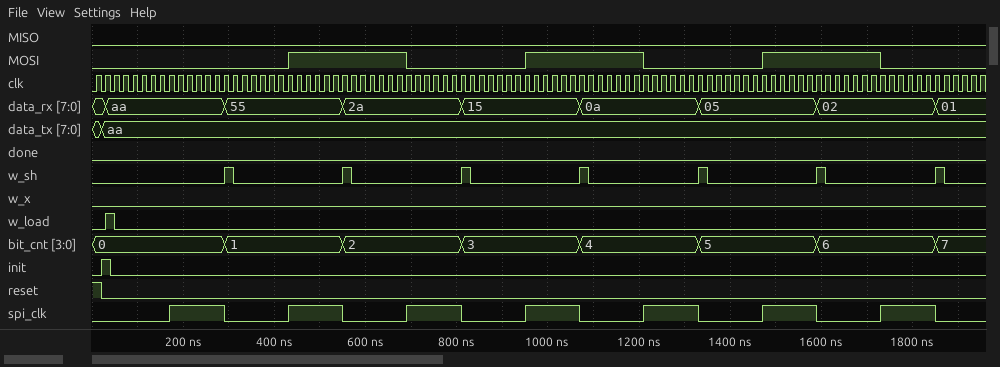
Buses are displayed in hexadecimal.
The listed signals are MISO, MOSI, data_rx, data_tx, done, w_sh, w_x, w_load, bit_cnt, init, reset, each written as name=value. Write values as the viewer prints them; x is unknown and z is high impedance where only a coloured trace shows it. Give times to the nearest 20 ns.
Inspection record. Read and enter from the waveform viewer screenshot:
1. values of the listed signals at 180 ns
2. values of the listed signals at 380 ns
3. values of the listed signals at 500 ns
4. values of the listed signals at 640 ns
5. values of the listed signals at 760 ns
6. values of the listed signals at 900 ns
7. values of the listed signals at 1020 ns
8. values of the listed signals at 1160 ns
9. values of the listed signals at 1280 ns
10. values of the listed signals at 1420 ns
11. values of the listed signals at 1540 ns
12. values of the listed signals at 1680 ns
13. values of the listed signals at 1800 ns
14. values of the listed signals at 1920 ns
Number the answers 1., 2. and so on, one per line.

1. MISO=0, MOSI=0, data_rx=aa, data_tx=aa, done=0, w_sh=0, w_x=0, w_load=0, bit_cnt=0, init=0, reset=0
2. MISO=0, MOSI=0, data_rx=55, data_tx=aa, done=0, w_sh=0, w_x=0, w_load=0, bit_cnt=1, init=0, reset=0
3. MISO=0, MOSI=1, data_rx=55, data_tx=aa, done=0, w_sh=0, w_x=0, w_load=0, bit_cnt=1, init=0, reset=0
4. MISO=0, MOSI=1, data_rx=2a, data_tx=aa, done=0, w_sh=0, w_x=0, w_load=0, bit_cnt=2, init=0, reset=0
5. MISO=0, MOSI=0, data_rx=2a, data_tx=aa, done=0, w_sh=0, w_x=0, w_load=0, bit_cnt=2, init=0, reset=0
6. MISO=0, MOSI=0, data_rx=15, data_tx=aa, done=0, w_sh=0, w_x=0, w_load=0, bit_cnt=3, init=0, reset=0
7. MISO=0, MOSI=1, data_rx=15, data_tx=aa, done=0, w_sh=0, w_x=0, w_load=0, bit_cnt=3, init=0, reset=0
8. MISO=0, MOSI=1, data_rx=0a, data_tx=aa, done=0, w_sh=0, w_x=0, w_load=0, bit_cnt=4, init=0, reset=0
9. MISO=0, MOSI=0, data_rx=0a, data_tx=aa, done=0, w_sh=0, w_x=0, w_load=0, bit_cnt=4, init=0, reset=0
10. MISO=0, MOSI=0, data_rx=05, data_tx=aa, done=0, w_sh=0, w_x=0, w_load=0, bit_cnt=5, init=0, reset=0
11. MISO=0, MOSI=1, data_rx=05, data_tx=aa, done=0, w_sh=0, w_x=0, w_load=0, bit_cnt=5, init=0, reset=0
12. MISO=0, MOSI=1, data_rx=02, data_tx=aa, done=0, w_sh=0, w_x=0, w_load=0, bit_cnt=6, init=0, reset=0
13. MISO=0, MOSI=0, data_rx=02, data_tx=aa, done=0, w_sh=0, w_x=0, w_load=0, bit_cnt=6, init=0, reset=0
14. MISO=0, MOSI=0, data_rx=01, data_tx=aa, done=0, w_sh=0, w_x=0, w_load=0, bit_cnt=7, init=0, reset=0
